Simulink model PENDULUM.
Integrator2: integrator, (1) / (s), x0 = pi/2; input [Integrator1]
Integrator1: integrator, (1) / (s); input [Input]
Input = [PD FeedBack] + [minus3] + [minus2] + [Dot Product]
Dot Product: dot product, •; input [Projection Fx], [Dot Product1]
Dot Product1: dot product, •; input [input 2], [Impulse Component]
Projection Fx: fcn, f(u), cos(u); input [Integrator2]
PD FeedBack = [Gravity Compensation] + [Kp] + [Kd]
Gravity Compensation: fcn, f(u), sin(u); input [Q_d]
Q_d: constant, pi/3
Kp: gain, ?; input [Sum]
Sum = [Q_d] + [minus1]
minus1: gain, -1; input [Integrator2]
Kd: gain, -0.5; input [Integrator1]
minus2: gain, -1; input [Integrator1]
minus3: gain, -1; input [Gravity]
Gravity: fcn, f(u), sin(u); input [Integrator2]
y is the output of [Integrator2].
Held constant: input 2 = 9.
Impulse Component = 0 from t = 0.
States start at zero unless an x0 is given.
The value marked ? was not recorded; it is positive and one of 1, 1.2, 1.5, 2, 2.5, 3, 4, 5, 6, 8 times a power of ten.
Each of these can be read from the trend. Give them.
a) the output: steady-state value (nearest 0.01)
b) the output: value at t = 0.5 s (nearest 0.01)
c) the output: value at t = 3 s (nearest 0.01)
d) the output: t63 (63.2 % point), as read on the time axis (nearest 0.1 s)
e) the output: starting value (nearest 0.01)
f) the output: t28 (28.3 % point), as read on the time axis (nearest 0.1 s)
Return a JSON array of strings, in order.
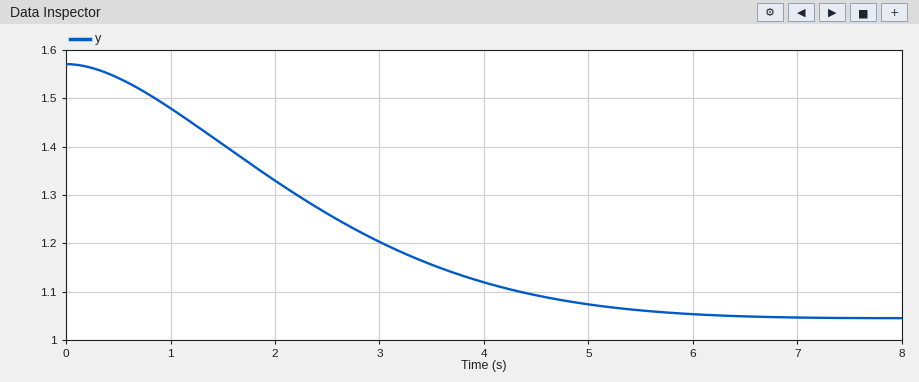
["1.05", "1.54", "1.20", "2.7 s", "1.57", "1.4 s"]
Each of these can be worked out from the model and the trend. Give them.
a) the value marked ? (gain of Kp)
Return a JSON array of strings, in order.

["0.3"]
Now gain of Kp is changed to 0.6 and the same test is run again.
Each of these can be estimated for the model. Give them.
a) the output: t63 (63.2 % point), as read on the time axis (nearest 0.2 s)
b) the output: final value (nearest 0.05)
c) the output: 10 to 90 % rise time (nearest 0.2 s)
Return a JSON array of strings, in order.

["2.0 s", "1.05", "2.4 s"]
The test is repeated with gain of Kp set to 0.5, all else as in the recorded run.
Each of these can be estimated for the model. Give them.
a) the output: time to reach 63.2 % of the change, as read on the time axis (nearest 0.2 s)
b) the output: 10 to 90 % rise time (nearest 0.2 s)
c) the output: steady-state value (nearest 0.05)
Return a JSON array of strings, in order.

["2.2 s", "2.8 s", "1.05"]
